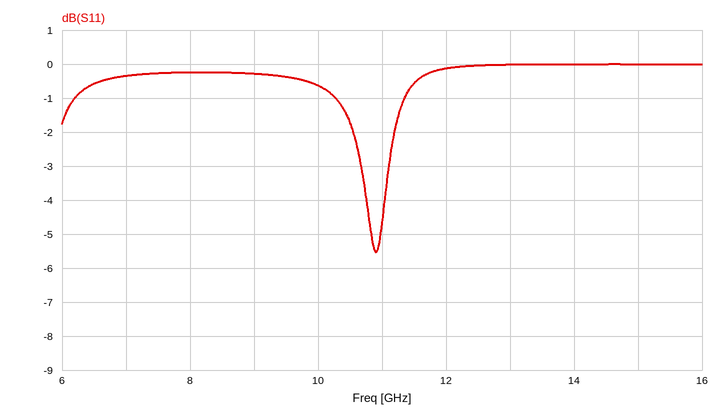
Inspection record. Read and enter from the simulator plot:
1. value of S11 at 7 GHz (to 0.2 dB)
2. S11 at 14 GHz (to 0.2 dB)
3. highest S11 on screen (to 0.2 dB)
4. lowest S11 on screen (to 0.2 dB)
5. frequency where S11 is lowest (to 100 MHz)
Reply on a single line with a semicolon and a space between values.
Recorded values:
-0.4 dB; 0.0 dB; 0.0 dB; -5.6 dB; 10.9 GHz
